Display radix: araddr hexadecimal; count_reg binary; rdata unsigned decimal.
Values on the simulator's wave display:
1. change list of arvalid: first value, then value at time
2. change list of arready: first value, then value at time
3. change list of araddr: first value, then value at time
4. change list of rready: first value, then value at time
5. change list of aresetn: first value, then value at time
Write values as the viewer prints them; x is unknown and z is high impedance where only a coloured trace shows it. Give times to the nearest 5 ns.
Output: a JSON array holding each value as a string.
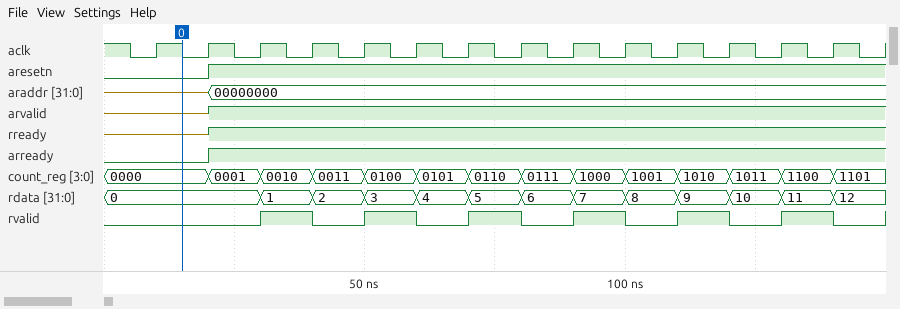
["z, 1 at 20 ns", "0, 1 at 20 ns", "z, 00000000 at 20 ns", "z, 1 at 20 ns", "0, 1 at 20 ns"]
